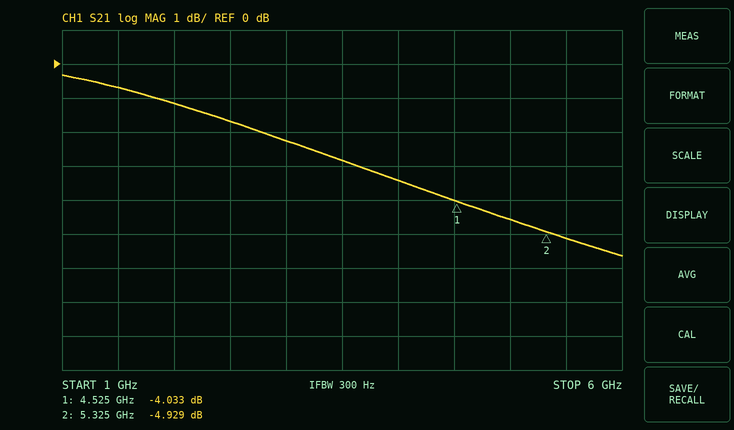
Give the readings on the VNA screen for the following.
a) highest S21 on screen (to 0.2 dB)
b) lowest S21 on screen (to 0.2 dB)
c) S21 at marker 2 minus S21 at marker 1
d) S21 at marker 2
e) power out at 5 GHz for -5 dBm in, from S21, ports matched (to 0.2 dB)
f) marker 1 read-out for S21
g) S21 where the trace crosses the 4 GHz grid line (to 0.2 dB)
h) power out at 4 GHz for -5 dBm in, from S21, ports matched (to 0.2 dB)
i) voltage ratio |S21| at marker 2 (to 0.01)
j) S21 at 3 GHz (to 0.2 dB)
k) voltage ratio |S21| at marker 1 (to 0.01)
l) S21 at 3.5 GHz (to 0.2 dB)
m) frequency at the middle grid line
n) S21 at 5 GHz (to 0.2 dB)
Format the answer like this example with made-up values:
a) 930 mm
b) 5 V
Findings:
a) -0.4 dB
b) -5.6 dB
c) -0.896 dB
d) -4.929 dB
e) -9.6 dBm
f) -4.033 dB
g) -3.4 dB
h) -8.4 dBm
i) 0.57
j) -2.2 dB
k) 0.63
l) -2.8 dB
m) 3.5 GHz
n) -4.6 dB
